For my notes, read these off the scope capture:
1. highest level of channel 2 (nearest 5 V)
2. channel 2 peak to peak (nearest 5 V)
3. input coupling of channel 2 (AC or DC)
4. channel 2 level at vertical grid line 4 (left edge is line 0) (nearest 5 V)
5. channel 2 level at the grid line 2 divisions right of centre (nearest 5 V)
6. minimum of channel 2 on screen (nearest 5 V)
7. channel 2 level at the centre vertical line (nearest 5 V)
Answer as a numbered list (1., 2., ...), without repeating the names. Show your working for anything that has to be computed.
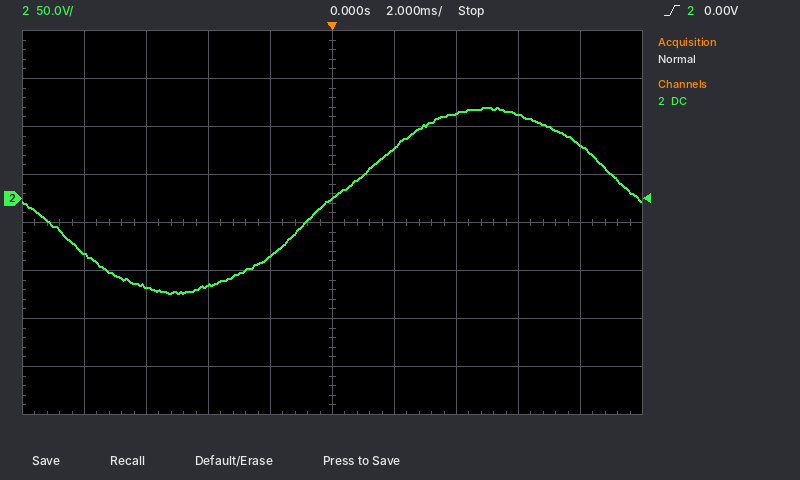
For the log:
1. 95 V
2. 95 V − (-100 V) = 195 V
3. DC
4. -60 V
5. 90 V
6. -100 V
7. 0 V
